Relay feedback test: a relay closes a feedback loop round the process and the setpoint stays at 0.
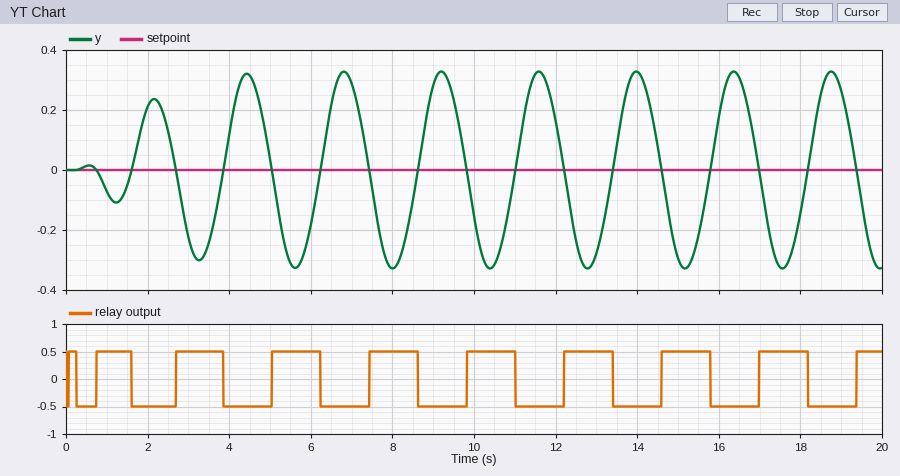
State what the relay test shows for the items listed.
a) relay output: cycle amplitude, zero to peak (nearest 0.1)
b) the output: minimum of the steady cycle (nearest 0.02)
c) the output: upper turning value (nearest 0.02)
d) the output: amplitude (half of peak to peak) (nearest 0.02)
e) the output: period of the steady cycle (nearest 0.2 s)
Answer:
0.5
-0.32
0.32
0.32
2.4 s
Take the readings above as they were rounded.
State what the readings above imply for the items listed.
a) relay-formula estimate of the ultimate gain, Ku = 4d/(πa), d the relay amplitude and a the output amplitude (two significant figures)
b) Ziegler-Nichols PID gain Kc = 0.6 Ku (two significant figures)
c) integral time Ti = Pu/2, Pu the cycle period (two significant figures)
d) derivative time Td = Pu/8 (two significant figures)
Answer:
2.0
1.2
1.2 s
0.30 s
